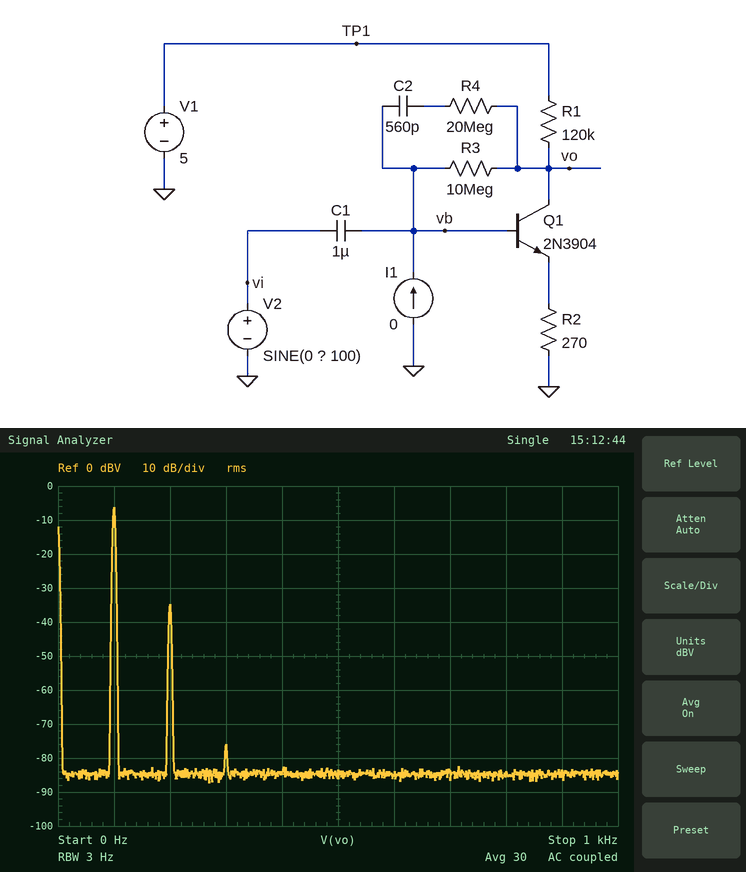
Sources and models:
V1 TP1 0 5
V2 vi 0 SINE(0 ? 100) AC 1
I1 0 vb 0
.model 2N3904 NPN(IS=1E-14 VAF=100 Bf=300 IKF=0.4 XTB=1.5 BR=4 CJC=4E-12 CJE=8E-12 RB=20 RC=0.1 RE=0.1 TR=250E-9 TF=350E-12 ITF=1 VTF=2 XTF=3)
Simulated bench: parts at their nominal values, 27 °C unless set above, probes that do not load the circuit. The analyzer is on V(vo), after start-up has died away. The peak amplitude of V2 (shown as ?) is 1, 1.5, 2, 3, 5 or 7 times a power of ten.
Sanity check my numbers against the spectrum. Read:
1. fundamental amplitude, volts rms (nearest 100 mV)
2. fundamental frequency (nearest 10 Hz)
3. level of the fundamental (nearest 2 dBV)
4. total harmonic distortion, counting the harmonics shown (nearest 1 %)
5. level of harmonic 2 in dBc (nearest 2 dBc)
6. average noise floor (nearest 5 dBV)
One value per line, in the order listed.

500 mV
100 Hz
-6 dBV
4 %
-28 dBc
-85 dBV
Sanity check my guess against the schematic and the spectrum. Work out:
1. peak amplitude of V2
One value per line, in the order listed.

7 mV
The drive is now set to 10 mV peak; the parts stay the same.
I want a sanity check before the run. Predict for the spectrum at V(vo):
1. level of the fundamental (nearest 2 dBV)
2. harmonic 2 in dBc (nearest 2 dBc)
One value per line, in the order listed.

-4 dBV
-26 dBc
